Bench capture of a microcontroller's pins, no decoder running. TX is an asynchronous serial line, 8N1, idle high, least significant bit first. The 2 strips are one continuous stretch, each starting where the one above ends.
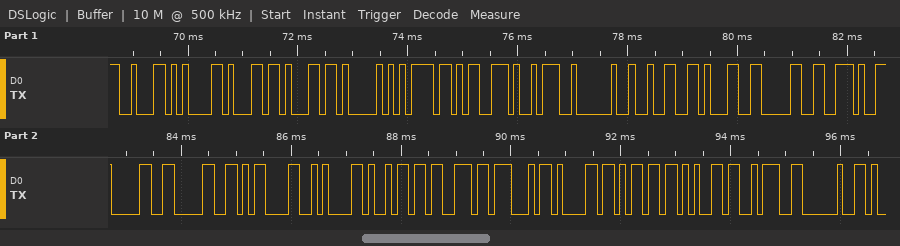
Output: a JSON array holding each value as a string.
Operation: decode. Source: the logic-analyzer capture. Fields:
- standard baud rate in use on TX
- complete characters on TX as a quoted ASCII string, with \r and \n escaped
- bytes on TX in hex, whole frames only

["9600 baud", "\"ballPos: 210.00\\r\\nisGame: \"", "62 61 6C 6C 50 6F 73 3A 20 32 31 30 2E 30 30 0D 0A 69 73 47 61 6D 65 3A 20"]
